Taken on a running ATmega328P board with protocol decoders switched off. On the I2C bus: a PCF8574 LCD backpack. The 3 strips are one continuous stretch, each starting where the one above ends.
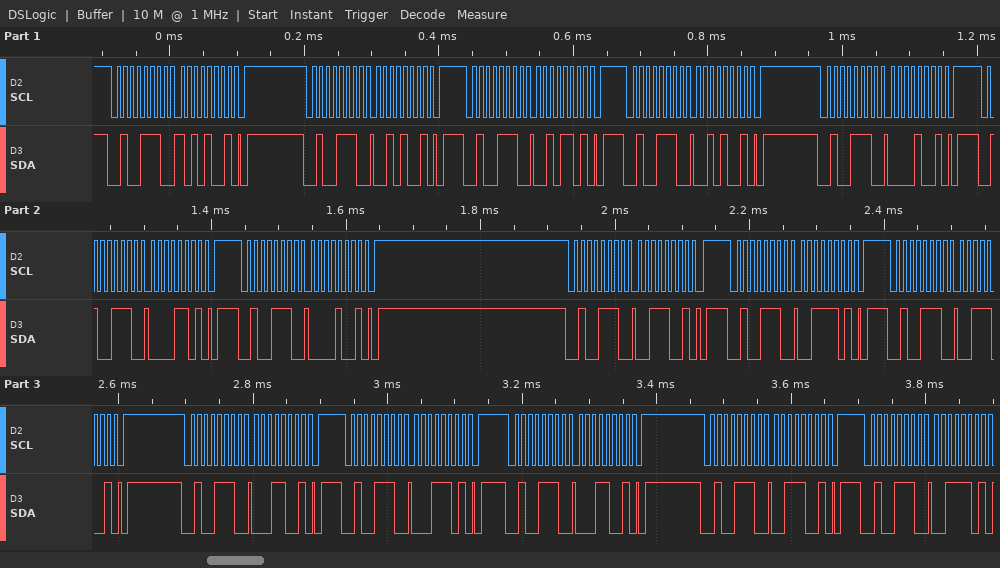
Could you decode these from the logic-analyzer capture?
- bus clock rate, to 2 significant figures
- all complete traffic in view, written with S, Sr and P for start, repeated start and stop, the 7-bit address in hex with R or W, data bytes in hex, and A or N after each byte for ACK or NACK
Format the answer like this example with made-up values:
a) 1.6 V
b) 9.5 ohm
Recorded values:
a) 100 kHz
b) S 27W A A9 A P S 27W A 29 A P S 27W A 2D A P S 27W A 29 A P S 27W A 09 A P S 27W A 0D A P S 27W A 09 A P S 27W A 39 A P S 27W A 3D A P S 27W A 39 A P S 27W A 19 A P S 27W A 1D A P S 27W A 19 A P S 27W A 39 A P S 27W A 3D A
